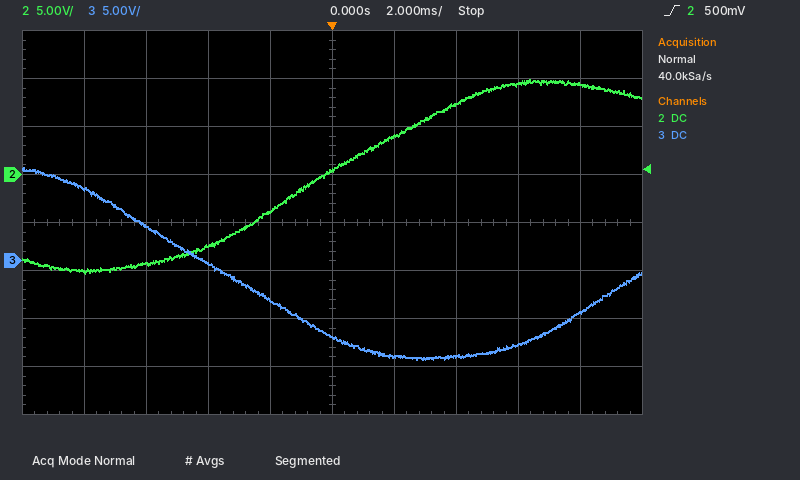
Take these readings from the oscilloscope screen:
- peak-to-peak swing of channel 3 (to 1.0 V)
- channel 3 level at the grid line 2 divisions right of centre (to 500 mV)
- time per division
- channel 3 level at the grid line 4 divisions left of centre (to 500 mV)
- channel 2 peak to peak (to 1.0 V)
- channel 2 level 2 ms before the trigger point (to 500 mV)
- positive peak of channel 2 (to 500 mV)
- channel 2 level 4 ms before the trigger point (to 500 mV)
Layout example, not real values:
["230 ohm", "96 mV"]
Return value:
["20.0 V", "-10.0 V", "2 ms", "7.5 V", "20.0 V", "-4.0 V", "10.0 V", "-7.5 V"]
